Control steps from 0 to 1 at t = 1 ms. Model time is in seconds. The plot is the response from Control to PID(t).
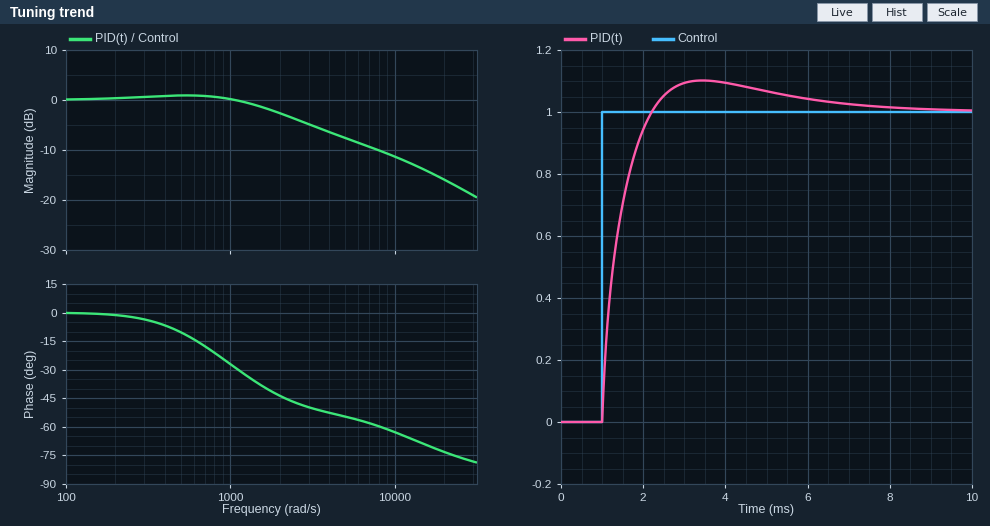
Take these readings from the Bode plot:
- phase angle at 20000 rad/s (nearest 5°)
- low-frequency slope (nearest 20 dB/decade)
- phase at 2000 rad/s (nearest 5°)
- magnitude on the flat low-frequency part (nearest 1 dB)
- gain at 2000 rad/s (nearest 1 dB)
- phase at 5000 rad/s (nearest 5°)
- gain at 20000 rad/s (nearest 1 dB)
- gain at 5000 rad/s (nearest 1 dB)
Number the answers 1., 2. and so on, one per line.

1. -75°
2. 0 dB/decade
3. -45°
4. 0 dB
5. -3 dB
6. -55°
7. -16 dB
8. -8 dB
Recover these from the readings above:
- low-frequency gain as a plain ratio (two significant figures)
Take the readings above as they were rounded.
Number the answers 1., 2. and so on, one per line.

1. 1.0
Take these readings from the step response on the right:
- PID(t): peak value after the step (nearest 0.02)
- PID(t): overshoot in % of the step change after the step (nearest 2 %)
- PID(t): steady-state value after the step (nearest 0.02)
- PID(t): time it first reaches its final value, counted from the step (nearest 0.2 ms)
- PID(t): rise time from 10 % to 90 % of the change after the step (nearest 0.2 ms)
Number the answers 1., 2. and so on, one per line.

1. 1.10
2. 10 %
3. 1.00
4. 1.2 ms
5. 0.8 ms
